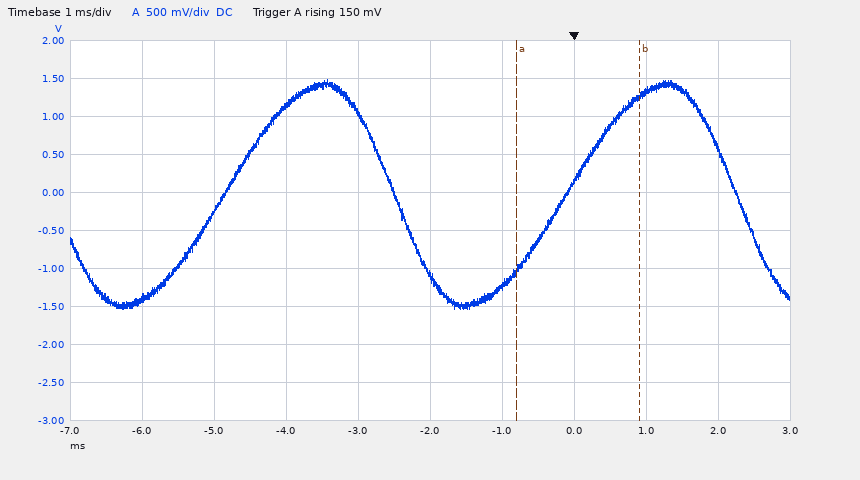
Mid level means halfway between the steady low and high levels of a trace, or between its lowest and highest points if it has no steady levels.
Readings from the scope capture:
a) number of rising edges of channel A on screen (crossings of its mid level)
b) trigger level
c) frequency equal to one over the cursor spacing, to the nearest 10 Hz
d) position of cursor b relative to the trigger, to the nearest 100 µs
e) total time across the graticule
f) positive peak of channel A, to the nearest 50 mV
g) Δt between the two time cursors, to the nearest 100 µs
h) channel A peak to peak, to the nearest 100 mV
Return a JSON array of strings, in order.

["2", "150 mV", "590 Hz", "+900 µs", "10 ms", "1.50 V", "1.7 ms", "3.00 V"]
